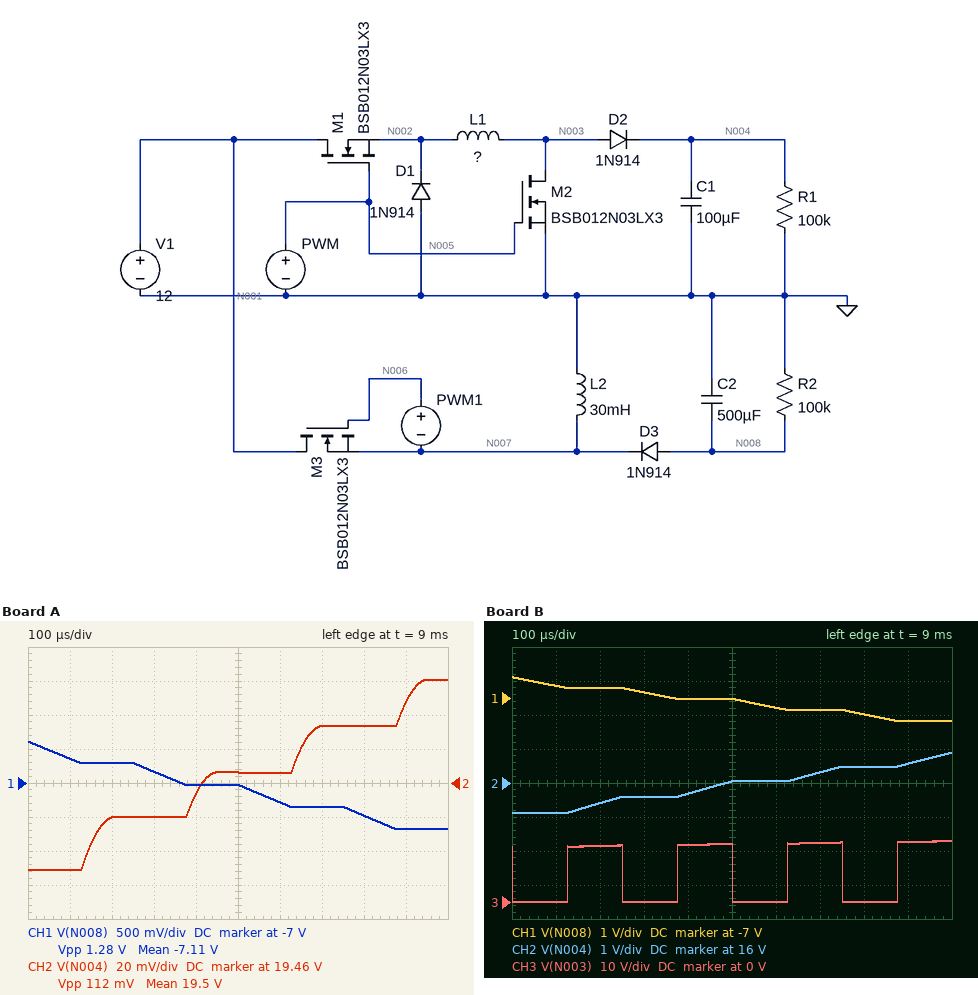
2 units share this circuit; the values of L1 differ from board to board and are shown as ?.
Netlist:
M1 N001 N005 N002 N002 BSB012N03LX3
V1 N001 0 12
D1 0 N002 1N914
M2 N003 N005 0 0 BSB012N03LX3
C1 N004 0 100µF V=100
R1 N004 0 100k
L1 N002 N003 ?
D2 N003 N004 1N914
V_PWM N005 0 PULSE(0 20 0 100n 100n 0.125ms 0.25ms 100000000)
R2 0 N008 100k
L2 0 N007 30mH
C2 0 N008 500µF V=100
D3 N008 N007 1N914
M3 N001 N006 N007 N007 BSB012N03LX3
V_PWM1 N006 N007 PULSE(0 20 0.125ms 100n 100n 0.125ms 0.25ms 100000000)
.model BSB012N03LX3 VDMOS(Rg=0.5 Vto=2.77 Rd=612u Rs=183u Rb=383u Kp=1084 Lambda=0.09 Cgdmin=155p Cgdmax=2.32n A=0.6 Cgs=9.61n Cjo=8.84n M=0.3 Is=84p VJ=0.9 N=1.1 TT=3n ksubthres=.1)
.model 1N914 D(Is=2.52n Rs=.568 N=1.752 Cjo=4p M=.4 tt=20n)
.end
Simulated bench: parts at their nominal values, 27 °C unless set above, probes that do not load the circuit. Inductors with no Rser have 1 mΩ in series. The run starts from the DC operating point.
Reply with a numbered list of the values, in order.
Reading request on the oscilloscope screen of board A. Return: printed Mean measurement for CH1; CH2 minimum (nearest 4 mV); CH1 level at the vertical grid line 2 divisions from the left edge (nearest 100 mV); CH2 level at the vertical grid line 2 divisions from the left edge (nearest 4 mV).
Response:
1. -7.11 V
2. 19.408 V
3. -6.7 V
4. 19.440 V
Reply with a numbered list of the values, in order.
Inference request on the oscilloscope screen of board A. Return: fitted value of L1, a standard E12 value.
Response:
1. 22 mH
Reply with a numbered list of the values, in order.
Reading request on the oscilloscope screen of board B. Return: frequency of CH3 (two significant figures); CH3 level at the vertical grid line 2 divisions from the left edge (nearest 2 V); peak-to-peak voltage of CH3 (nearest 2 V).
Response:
1. 4.0 kHz
2. 16 V
3. 18 V
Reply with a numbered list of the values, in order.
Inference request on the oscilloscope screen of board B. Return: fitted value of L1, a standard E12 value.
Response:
1. 47 mH
